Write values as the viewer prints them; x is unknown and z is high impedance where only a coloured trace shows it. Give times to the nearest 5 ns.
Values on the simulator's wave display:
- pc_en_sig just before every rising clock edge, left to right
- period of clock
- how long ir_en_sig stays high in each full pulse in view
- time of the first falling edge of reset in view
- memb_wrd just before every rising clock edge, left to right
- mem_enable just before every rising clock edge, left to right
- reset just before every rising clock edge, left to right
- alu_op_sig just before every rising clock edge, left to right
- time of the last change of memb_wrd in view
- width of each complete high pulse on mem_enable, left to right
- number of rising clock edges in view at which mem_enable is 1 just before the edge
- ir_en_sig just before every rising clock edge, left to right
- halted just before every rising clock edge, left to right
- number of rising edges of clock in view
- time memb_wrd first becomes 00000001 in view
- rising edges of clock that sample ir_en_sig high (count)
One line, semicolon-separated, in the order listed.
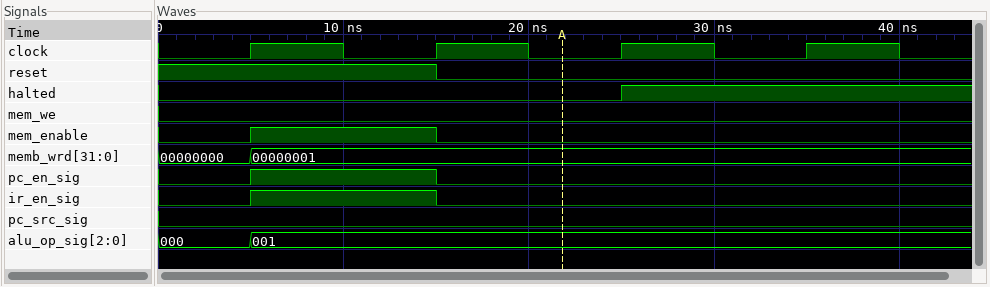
0 1 0 0; 10 ns; 10 ns; 15 ns; 00000000, 00000001, 00000001, 00000001; 0 1 0 0; 1 1 0 0; 000, 001, 001, 001; 5 ns; 10 ns; 1; 0 1 0 0; 0 0 0 1; 4; 5 ns; 1
